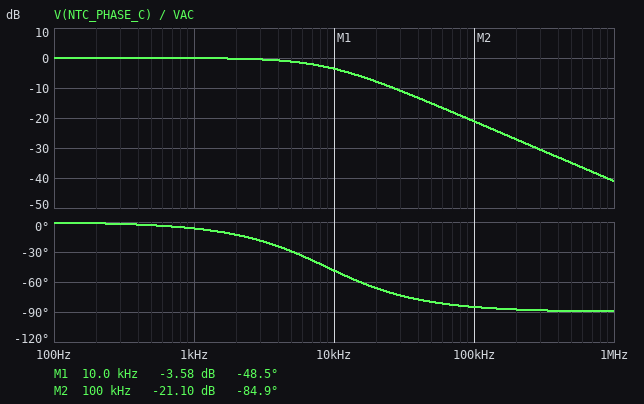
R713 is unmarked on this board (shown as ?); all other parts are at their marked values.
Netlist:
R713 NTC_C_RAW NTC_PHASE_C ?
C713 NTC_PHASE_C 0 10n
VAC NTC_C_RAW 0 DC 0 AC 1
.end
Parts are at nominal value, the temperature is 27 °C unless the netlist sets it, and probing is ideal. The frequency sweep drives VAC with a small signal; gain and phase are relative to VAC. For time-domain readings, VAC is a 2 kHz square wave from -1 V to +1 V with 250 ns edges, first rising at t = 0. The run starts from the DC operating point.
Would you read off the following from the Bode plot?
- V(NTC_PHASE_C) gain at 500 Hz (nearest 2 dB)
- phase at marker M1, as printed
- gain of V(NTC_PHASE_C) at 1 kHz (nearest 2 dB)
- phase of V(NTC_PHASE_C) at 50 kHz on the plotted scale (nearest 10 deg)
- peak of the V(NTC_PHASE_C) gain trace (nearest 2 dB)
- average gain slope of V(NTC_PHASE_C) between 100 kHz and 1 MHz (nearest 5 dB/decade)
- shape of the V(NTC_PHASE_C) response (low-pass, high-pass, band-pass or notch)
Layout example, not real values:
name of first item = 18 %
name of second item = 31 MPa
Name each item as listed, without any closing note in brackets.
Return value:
V(NTC_PHASE_C) gain at 500 Hz = 0 dB
phase at marker M1, as printed = -48.5 deg
gain of V(NTC_PHASE_C) at 1 kHz = 0 dB
phase of V(NTC_PHASE_C) at 50 kHz on the plotted scale = -80 deg
peak of the V(NTC_PHASE_C) gain trace = 0 dB
average gain slope of V(NTC_PHASE_C) between 100 kHz and 1 MHz = -20 dB/decade
shape of the V(NTC_PHASE_C) response = low-pass
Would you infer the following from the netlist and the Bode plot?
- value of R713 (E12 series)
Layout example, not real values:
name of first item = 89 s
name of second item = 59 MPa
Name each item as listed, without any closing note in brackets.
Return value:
value of R713 = 1.8 kΩ
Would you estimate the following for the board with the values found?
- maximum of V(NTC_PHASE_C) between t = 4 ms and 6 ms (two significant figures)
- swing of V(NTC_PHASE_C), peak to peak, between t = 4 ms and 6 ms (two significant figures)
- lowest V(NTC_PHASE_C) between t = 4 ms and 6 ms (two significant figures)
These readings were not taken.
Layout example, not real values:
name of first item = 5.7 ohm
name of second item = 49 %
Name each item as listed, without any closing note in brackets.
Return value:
maximum of V(NTC_PHASE_C) between t = 4 ms and 6 ms = 1.0 V
swing of V(NTC_PHASE_C), peak to peak, between t = 4 ms and 6 ms = 2.0 V
lowest V(NTC_PHASE_C) between t = 4 ms and 6 ms = -1.0 V
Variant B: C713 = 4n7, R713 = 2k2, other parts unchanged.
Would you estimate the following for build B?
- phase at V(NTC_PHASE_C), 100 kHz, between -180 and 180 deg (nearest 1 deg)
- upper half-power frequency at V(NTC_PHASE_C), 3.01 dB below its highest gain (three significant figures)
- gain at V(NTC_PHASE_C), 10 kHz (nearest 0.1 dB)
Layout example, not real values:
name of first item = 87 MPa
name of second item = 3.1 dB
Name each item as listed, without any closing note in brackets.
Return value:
phase at V(NTC_PHASE_C), 100 kHz, between -180 and 180 deg = -81 deg
upper half-power frequency at V(NTC_PHASE_C), 3.01 dB below its highest gain = 15.4 kHz
gain at V(NTC_PHASE_C), 10 kHz = -1.5 dB
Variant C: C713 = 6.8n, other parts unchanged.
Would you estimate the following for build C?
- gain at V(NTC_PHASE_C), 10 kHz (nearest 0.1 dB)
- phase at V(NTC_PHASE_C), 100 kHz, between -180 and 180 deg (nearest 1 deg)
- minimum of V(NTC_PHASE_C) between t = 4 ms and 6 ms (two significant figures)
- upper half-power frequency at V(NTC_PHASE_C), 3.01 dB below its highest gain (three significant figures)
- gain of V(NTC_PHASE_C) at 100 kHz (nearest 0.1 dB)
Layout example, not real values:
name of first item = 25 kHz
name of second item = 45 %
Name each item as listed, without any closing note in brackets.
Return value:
gain at V(NTC_PHASE_C), 10 kHz = -2.0 dB
phase at V(NTC_PHASE_C), 100 kHz, between -180 and 180 deg = -83 deg
minimum of V(NTC_PHASE_C) between t = 4 ms and 6 ms = -1.0 V
upper half-power frequency at V(NTC_PHASE_C), 3.01 dB below its highest gain = 13.0 kHz
gain of V(NTC_PHASE_C) at 100 kHz = -17.8 dB
